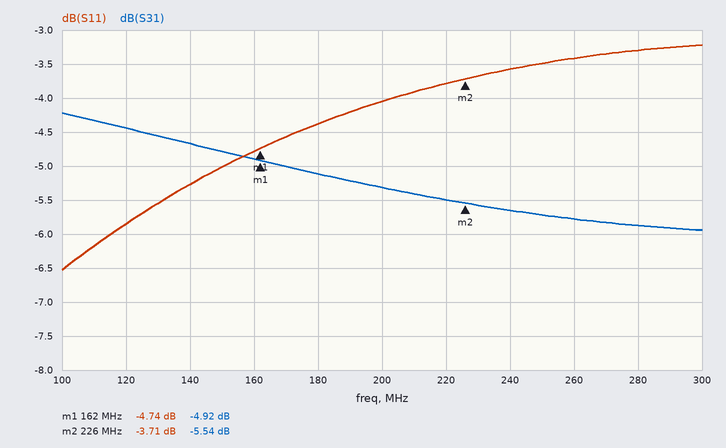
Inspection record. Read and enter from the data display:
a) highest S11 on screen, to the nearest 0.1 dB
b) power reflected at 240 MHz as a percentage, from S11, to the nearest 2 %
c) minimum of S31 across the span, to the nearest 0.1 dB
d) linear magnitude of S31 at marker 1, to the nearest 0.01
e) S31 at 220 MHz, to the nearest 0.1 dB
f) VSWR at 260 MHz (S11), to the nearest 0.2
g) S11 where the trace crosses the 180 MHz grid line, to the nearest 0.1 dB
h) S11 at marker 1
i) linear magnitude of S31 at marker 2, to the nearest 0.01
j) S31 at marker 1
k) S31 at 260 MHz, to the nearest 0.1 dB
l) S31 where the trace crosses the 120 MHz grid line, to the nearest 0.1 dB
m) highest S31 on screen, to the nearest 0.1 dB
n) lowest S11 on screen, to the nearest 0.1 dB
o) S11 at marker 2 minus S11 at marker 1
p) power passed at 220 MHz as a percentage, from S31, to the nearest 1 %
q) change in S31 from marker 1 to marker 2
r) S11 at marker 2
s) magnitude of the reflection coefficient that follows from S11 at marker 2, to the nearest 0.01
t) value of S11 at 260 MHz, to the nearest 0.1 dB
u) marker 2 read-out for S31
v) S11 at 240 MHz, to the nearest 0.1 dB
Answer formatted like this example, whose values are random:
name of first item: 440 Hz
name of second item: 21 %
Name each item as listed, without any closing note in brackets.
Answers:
highest S11 on screen, to the nearest 0.1 dB: -3.2 dB
power reflected at 240 MHz as a percentage, from S11, to the nearest 2 %: 44 %
minimum of S31 across the span, to the nearest 0.1 dB: -5.9 dB
linear magnitude of S31 at marker 1, to the nearest 0.01: 0.57
S31 at 220 MHz, to the nearest 0.1 dB: -5.5 dB
VSWR at 260 MHz (S11), to the nearest 0.2: 5.2
S11 where the trace crosses the 180 MHz grid line, to the nearest 0.1 dB: -4.4 dB
S11 at marker 1: -4.74 dB
linear magnitude of S31 at marker 2, to the nearest 0.01: 0.53
S31 at marker 1: -4.92 dB
S31 at 260 MHz, to the nearest 0.1 dB: -5.8 dB
S31 where the trace crosses the 120 MHz grid line, to the nearest 0.1 dB: -4.4 dB
highest S31 on screen, to the nearest 0.1 dB: -4.2 dB
lowest S11 on screen, to the nearest 0.1 dB: -6.5 dB
S11 at marker 2 minus S11 at marker 1: 1.03 dB
power passed at 220 MHz as a percentage, from S31, to the nearest 1 %: 28 %
change in S31 from marker 1 to marker 2: -0.62 dB
S11 at marker 2: -3.71 dB
magnitude of the reflection coefficient that follows from S11 at marker 2, to the nearest 0.01: 0.65
value of S11 at 260 MHz, to the nearest 0.1 dB: -3.4 dB
marker 2 read-out for S31: -5.54 dB
S11 at 240 MHz, to the nearest 0.1 dB: -3.6 dB
